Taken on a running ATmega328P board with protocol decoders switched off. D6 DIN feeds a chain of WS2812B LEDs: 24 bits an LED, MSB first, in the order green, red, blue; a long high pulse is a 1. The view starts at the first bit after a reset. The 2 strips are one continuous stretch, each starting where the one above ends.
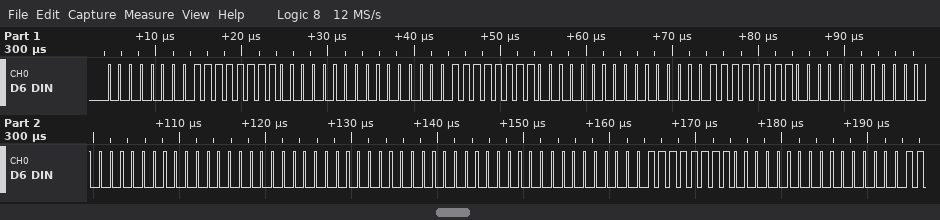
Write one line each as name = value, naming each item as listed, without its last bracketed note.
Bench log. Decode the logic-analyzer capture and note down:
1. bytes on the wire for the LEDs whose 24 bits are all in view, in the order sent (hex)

bytes on the wire for the LEDs whose 24 bits are all in view, in the order sent = 00 FF 00 00 FF 00 00 FF 00 00 00 00 00 00 00 00 FF 00
